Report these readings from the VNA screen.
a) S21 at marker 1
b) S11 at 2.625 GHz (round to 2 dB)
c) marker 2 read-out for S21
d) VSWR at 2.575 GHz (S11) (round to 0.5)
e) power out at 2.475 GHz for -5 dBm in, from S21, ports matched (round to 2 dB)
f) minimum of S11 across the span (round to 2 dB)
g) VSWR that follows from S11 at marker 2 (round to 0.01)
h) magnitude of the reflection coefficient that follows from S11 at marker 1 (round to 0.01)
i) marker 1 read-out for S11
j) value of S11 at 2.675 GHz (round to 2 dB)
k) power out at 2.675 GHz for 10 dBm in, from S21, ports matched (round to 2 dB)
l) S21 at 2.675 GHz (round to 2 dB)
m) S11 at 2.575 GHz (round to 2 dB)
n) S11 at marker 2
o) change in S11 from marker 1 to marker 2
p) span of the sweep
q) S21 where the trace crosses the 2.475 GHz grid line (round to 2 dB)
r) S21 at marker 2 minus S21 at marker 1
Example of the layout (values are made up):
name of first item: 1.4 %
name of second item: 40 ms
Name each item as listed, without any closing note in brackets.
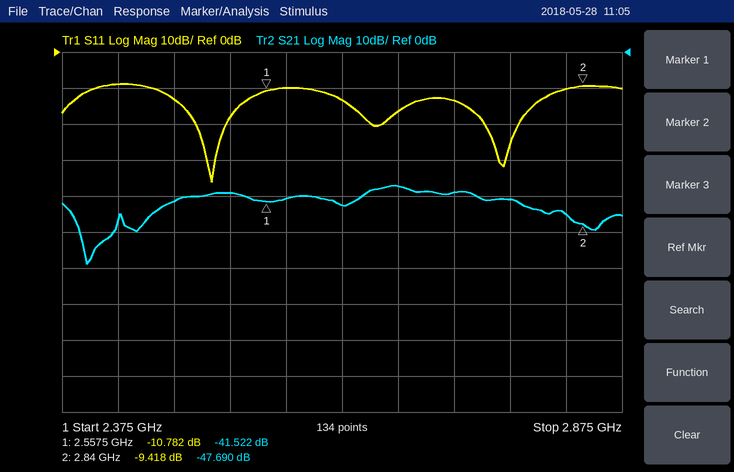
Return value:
S21 at marker 1: -41.522 dB
S11 at 2.625 GHz: -14 dB
marker 2 read-out for S21: -47.690 dB
VSWR at 2.575 GHz (S11): 2.0
power out at 2.475 GHz for -5 dBm in, from S21, ports matched: -46 dBm
minimum of S11 across the span: -36 dB
VSWR that follows from S11 at marker 2: 2.02
magnitude of the reflection coefficient that follows from S11 at marker 1: 0.29
marker 1 read-out for S11: -10.782 dB
value of S11 at 2.675 GHz: -16 dB
power out at 2.675 GHz for 10 dBm in, from S21, ports matched: -28 dBm
S21 at 2.675 GHz: -38 dB
S11 at 2.575 GHz: -10 dB
S11 at marker 2: -9.418 dB
change in S11 from marker 1 to marker 2: 1.364 dB
span of the sweep: 500 MHz
S21 where the trace crosses the 2.475 GHz grid line: -42 dB
S21 at marker 2 minus S21 at marker 1: -6.168 dB
